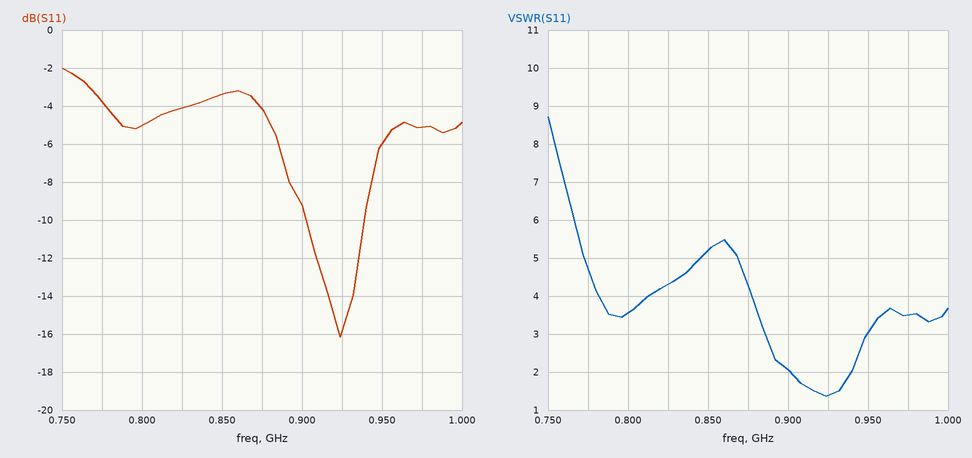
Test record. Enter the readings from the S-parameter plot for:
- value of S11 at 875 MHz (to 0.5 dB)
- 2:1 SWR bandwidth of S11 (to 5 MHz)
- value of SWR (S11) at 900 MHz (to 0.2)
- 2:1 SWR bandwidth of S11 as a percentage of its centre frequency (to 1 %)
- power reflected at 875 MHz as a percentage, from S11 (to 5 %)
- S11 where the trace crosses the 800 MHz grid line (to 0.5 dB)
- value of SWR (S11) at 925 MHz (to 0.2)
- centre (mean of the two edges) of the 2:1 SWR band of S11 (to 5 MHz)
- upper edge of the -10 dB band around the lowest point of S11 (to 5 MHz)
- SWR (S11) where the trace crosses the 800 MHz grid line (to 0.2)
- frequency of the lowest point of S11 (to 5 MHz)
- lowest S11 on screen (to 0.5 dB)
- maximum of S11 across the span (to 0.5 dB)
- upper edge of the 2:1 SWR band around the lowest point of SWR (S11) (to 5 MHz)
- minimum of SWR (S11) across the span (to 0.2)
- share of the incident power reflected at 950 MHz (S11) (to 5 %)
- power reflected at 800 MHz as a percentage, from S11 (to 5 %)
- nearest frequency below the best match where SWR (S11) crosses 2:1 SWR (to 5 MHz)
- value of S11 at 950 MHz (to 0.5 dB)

-4.0 dB
40 MHz
2.0
4 %
40 %
-5.0 dB
1.4
920 MHz
940 MHz
3.6
925 MHz
-16.0 dB
-2.0 dB
940 MHz
1.4
25 %
30 %
900 MHz
-6.0 dB
